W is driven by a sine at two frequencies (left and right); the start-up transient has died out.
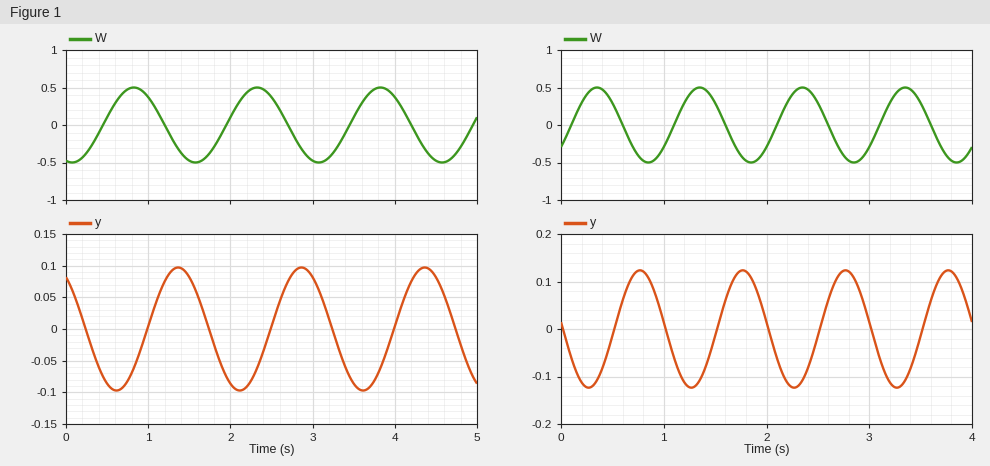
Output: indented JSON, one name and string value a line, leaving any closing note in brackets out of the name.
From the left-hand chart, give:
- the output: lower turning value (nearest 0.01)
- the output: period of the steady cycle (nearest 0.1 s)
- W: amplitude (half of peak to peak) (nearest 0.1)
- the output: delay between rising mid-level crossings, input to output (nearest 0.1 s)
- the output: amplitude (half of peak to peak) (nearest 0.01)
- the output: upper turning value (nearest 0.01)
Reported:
{
  "the output: lower turning value": "-0.10",
  "the output: period of the steady cycle": "1.5 s",
  "W: amplitude (half of peak to peak)": "0.5",
  "the output: delay between rising mid-level crossings, input to output": "0.5 s",
  "the output: amplitude (half of peak to peak)": "0.10",
  "the output: upper turning value": "0.10"
}
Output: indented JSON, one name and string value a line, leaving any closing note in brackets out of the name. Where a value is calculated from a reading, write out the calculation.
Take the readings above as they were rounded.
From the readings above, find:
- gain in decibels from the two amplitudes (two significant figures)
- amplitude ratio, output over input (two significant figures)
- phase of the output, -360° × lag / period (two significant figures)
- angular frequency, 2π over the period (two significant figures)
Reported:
{
  "gain in decibels from the two amplitudes": "20 log10(0.1 / 0.5) = -14 dB",
  "amplitude ratio, output over input": "0.1 / 0.5 = 0.20",
  "phase of the output, -360° × lag / period": "-360 × 0.5 / 1.5 = -120°",
  "angular frequency, 2π over the period": "2π / 1.5 = 4.2 rad/s"
}
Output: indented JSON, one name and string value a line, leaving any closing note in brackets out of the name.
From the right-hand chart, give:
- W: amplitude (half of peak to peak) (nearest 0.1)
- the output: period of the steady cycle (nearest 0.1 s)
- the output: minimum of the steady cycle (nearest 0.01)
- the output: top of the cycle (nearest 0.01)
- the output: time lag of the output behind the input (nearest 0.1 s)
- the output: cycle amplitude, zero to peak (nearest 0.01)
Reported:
{
  "W: amplitude (half of peak to peak)": "0.5",
  "the output: period of the steady cycle": "1.0 s",
  "the output: minimum of the steady cycle": "-0.12",
  "the output: top of the cycle": "0.12",
  "the output: time lag of the output behind the input": "0.4 s",
  "the output: cycle amplitude, zero to peak": "0.12"
}
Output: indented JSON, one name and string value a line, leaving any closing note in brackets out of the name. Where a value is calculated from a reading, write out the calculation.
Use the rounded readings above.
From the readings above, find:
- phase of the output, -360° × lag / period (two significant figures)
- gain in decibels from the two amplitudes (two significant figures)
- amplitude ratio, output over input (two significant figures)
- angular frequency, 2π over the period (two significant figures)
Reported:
{
  "phase of the output, -360° × lag / period": "-360 × 0.4 / 1 = -140°",
  "gain in decibels from the two amplitudes": "20 log10(0.12 / 0.5) = -12 dB",
  "amplitude ratio, output over input": "0.12 / 0.5 = 0.24",
  "angular frequency, 2π over the period": "2π / 1 = 6.3 rad/s"
}
